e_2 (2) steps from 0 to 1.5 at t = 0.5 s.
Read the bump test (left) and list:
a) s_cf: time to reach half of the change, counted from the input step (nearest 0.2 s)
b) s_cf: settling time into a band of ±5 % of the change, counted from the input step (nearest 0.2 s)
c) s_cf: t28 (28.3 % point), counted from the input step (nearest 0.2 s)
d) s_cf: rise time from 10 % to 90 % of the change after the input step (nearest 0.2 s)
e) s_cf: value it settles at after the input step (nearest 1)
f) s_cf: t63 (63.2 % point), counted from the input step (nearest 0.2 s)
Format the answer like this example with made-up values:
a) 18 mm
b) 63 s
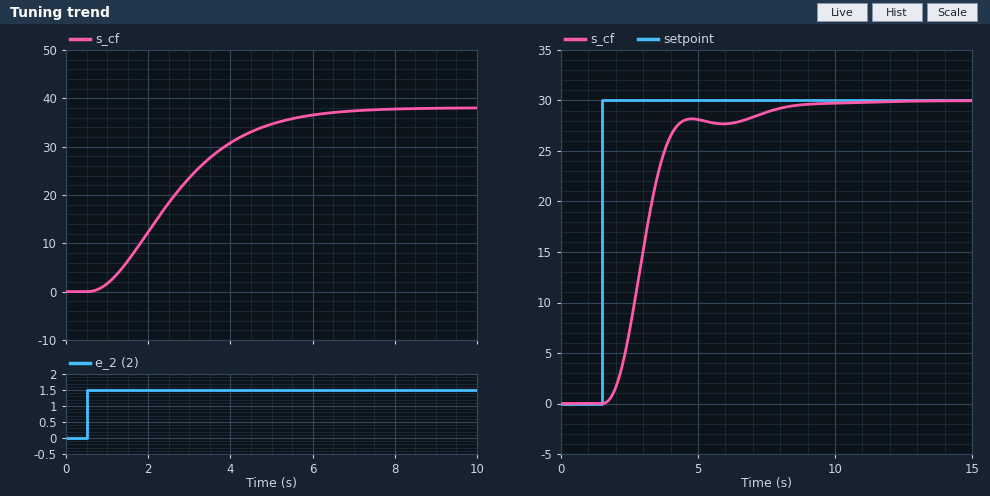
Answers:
a) 2.0 s
b) 5.2 s
c) 1.4 s
d) 3.6 s
e) 38
f) 2.6 s
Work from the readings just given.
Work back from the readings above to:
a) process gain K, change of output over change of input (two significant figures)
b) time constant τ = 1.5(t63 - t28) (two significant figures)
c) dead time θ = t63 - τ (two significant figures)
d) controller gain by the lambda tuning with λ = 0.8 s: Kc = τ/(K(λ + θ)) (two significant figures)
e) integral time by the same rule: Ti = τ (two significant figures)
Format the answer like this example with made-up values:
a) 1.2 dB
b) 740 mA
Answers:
a) 25
b) 1.8 s
c) 0.80 s
d) 0.045
e) 1.8 s
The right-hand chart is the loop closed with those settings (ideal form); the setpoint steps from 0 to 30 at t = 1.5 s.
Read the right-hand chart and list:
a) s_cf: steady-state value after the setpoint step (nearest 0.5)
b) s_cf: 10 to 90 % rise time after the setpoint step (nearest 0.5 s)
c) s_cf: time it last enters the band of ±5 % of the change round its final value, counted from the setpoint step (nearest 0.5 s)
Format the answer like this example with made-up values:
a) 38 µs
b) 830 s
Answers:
a) 30.0
b) 2.0 s
c) 5.5 s
